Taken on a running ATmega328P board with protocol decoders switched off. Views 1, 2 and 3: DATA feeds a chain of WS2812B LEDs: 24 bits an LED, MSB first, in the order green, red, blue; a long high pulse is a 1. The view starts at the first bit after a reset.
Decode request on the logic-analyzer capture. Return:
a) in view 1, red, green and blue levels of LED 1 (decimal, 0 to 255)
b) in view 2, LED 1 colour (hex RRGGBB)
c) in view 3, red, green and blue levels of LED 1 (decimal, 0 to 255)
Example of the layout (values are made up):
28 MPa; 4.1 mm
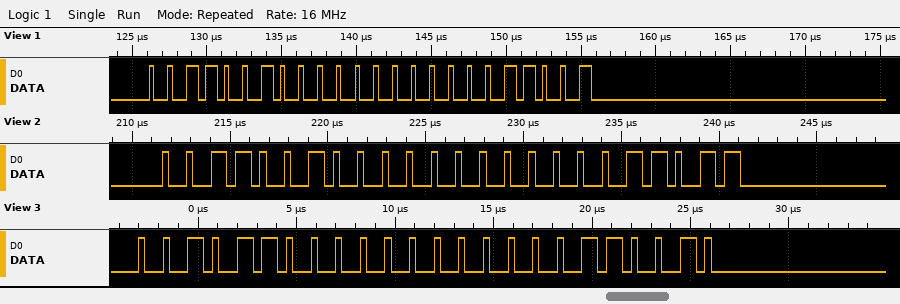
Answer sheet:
0, 50, 25; #00321B; 0, 44, 50
